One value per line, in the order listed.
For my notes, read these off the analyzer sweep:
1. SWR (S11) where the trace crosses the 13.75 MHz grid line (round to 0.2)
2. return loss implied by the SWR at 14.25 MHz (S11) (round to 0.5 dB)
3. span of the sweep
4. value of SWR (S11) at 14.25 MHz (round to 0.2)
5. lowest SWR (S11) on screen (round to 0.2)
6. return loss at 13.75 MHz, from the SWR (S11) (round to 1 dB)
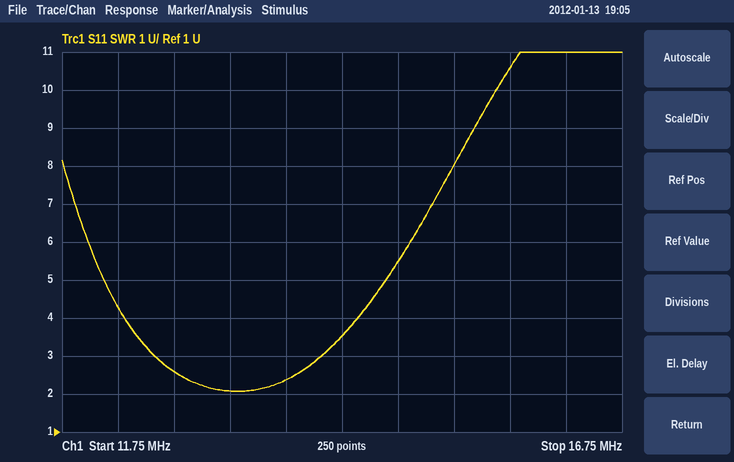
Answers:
2.4
5.0 dB
5 MHz
3.6
2.0
8 dB
